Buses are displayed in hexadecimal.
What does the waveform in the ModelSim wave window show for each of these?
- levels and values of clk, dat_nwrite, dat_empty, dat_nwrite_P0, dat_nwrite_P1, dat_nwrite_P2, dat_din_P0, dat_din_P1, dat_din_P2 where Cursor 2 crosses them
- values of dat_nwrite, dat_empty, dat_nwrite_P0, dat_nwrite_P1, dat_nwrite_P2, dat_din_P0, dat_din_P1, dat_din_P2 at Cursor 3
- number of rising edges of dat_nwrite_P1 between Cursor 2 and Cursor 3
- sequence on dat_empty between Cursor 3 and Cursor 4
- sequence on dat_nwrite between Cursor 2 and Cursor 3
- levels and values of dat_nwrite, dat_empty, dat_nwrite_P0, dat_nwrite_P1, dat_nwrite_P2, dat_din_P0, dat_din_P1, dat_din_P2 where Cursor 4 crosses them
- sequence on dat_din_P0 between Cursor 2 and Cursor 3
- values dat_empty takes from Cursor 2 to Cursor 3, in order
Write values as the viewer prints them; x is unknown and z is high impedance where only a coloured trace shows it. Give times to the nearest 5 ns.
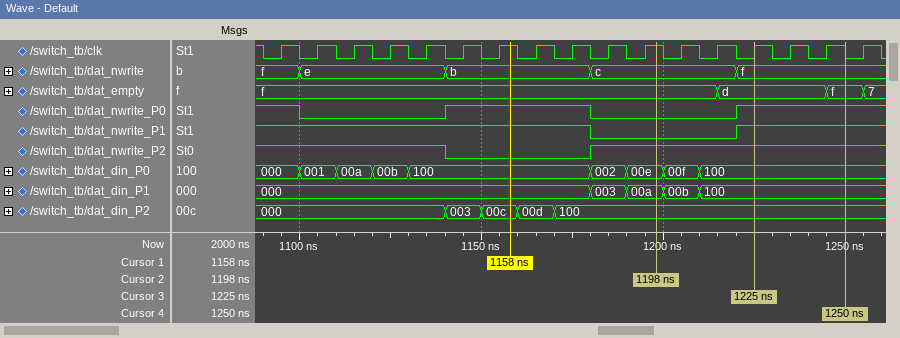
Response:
clk=1, dat_nwrite=c, dat_empty=f, dat_nwrite_P0=0, dat_nwrite_P1=0, dat_nwrite_P2=1, dat_din_P0=00e, dat_din_P1=00a, dat_din_P2=100
dat_nwrite=f, dat_empty=d, dat_nwrite_P0=1, dat_nwrite_P1=1, dat_nwrite_P2=1, dat_din_P0=100, dat_din_P1=100, dat_din_P2=100
1
d, f
c, f
dat_nwrite=f, dat_empty=f, dat_nwrite_P0=1, dat_nwrite_P1=1, dat_nwrite_P2=1, dat_din_P0=100, dat_din_P1=100, dat_din_P2=100
00e, 00f, 100
f, d
